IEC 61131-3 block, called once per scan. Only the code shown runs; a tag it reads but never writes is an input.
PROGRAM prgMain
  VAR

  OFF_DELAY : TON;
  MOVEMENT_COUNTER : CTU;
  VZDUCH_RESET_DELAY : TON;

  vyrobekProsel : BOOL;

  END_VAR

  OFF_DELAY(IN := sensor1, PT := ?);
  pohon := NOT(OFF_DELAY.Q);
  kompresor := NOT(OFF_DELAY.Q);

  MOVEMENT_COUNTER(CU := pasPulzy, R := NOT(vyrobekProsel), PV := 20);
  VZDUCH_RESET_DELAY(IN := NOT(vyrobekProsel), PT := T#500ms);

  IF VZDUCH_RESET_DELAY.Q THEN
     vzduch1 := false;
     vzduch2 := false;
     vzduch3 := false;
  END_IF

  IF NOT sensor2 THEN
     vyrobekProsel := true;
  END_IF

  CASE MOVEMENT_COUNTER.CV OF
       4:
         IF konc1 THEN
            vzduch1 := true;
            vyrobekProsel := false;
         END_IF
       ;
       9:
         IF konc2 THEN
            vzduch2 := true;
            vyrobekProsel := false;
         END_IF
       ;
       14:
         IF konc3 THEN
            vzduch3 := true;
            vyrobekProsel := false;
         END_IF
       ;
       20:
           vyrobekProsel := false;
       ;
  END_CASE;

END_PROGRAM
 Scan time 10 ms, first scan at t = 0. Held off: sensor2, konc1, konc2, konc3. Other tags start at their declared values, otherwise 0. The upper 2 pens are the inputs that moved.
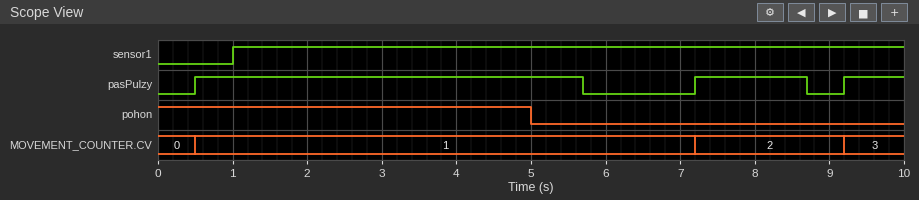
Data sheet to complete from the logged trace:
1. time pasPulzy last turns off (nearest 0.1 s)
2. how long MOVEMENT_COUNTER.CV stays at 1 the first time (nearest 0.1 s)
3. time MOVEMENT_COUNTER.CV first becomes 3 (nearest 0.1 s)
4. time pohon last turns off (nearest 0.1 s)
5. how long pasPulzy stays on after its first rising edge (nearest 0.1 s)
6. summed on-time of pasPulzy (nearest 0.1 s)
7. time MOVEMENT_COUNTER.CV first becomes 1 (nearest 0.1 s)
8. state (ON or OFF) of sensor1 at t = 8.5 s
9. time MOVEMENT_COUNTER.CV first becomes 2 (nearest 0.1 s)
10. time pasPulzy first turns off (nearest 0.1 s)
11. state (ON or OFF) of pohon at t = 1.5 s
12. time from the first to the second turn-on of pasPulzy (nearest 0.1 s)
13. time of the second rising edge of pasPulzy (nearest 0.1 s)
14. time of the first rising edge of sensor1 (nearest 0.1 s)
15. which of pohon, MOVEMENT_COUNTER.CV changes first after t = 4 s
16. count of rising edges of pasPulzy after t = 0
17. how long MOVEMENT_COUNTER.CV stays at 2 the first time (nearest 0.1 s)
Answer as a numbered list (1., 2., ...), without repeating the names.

1. 8.7 s
2. 6.7 s
3. 9.2 s
4. 5.0 s
5. 5.2 s
6. 7.5 s
7. 0.5 s
8. ON
9. 7.2 s
10. 5.7 s
11. ON
12. 6.7 s
13. 7.2 s
14. 1.0 s
15. pohon
16. 3
17. 2.0 s
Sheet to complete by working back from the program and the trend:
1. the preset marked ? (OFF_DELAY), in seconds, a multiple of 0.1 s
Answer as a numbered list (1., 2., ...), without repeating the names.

1. 4.0 s
